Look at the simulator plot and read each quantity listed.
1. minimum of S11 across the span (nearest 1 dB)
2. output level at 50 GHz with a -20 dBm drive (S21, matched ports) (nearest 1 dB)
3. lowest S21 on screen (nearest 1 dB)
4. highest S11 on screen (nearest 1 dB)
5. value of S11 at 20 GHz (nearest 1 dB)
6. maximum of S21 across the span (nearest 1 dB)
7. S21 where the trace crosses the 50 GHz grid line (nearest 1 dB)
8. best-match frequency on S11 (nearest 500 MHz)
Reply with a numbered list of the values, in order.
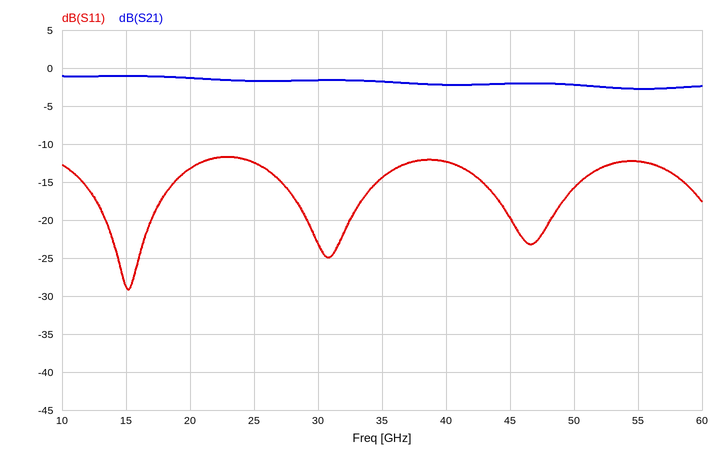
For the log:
1. -29 dB
2. -22 dBm
3. -3 dB
4. -12 dB
5. -13 dB
6. -1 dB
7. -2 dB
8. 15.0 GHz
